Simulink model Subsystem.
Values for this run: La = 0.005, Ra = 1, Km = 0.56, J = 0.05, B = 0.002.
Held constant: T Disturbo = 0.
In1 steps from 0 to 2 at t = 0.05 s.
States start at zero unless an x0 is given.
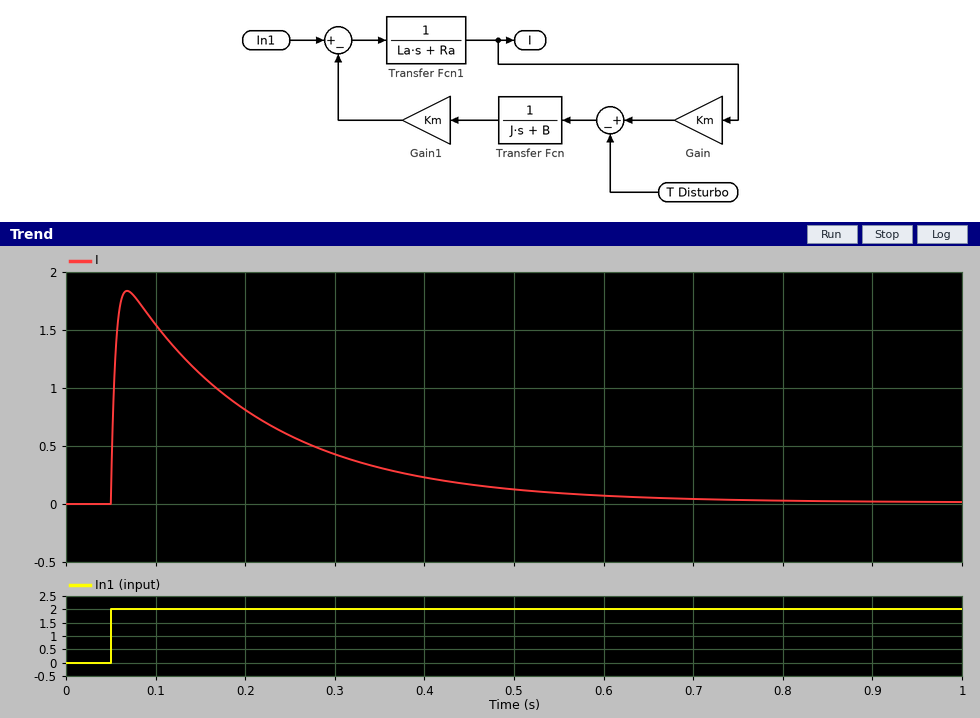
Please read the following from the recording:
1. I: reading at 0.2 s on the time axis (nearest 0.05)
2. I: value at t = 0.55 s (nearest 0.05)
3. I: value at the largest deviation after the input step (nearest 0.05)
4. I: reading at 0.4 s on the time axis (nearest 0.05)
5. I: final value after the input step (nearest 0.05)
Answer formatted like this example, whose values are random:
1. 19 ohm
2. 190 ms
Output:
1. 0.80
2. 0.10
3. 1.85
4. 0.25
5. 0.00
